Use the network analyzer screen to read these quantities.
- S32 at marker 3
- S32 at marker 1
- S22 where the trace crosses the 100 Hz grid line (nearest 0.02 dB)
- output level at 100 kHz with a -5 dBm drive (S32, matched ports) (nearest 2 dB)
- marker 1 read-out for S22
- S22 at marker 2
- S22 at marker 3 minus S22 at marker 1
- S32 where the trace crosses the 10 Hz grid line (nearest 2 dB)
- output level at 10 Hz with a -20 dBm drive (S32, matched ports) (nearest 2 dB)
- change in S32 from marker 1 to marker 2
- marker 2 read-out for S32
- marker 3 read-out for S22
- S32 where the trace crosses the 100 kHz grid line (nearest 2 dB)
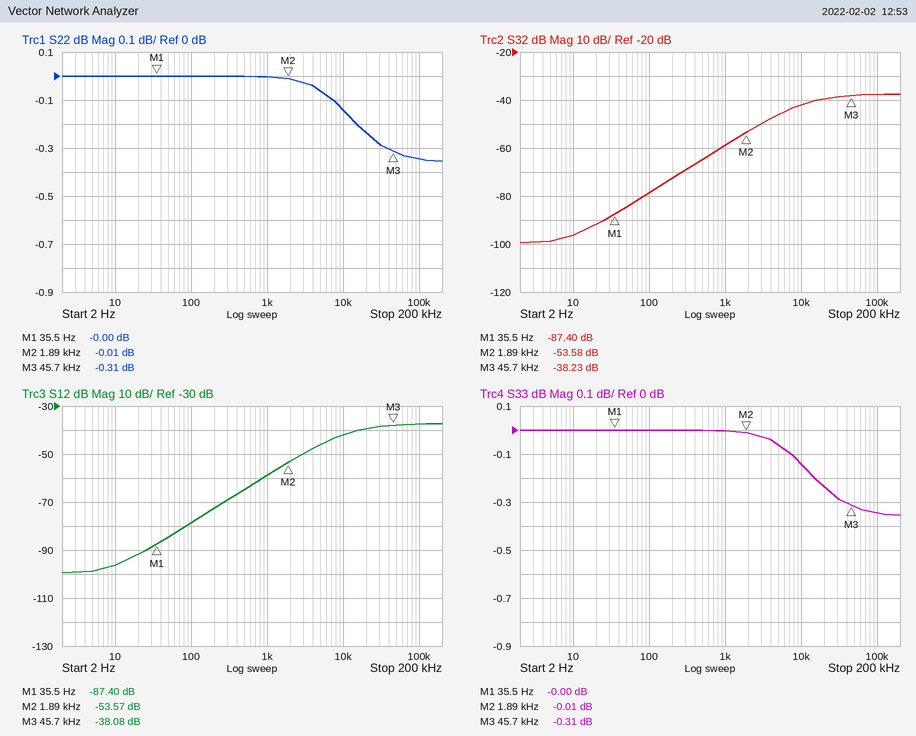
-38.23 dB
-87.40 dB
0.00 dB
-42 dBm
-0.00 dB
-0.01 dB
-0.31 dB
-96 dB
-116 dBm
33.82 dB
-53.58 dB
-0.31 dB
-38 dB
